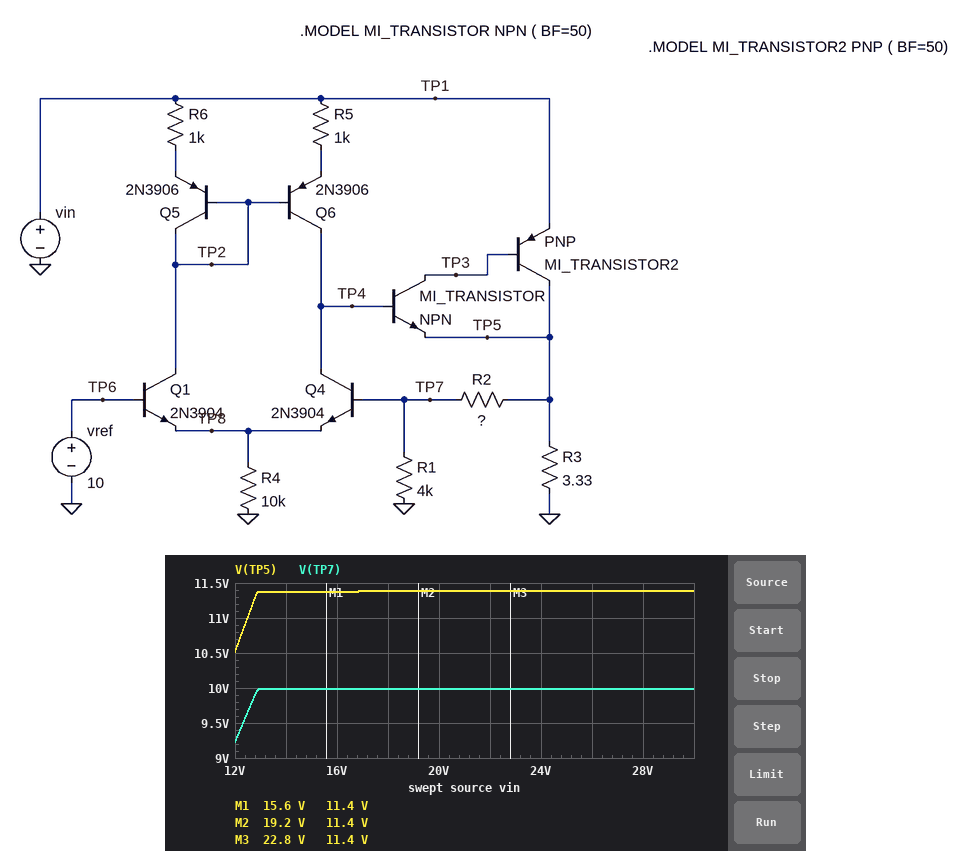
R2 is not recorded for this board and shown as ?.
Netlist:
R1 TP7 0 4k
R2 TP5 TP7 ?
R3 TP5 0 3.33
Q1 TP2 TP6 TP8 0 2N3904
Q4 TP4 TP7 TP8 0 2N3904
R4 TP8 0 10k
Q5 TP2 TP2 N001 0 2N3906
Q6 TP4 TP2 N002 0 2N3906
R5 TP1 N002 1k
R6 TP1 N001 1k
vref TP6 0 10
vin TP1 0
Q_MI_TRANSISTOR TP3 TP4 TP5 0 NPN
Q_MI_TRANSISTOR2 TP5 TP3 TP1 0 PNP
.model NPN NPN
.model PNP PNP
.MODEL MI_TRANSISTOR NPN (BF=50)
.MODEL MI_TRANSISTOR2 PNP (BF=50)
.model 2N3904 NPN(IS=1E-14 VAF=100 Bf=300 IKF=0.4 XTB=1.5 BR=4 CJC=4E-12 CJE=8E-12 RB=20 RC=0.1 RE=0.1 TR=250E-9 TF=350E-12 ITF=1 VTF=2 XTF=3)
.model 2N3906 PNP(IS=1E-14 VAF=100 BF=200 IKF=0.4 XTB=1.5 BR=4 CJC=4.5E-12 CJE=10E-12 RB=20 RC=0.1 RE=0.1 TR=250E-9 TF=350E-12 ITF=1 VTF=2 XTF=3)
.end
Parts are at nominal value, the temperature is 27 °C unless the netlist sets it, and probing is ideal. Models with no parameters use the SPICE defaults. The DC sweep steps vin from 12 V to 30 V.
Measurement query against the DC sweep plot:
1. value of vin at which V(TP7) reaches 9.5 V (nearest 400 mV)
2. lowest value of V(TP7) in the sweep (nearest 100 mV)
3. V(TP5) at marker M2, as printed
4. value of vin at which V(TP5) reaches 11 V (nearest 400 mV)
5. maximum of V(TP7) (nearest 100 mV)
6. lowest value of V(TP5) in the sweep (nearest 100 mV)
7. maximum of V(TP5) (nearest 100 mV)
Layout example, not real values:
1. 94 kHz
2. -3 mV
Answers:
1. 12.4 V
2. 9.2 V
3. 11.4 V
4. 12.4 V
5. 10.0 V
6. 10.5 V
7. 11.4 V
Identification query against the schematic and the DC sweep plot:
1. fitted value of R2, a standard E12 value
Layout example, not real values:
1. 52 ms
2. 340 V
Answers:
1. 560 Ω
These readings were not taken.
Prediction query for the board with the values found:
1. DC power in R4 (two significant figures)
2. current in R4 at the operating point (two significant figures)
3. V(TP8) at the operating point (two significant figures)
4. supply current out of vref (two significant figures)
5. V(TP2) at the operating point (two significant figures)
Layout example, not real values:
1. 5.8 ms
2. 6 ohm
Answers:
1. 8.6 mW
2. 930 µA
3. 9.3 V
4. 930 µA
5. 9.3 V
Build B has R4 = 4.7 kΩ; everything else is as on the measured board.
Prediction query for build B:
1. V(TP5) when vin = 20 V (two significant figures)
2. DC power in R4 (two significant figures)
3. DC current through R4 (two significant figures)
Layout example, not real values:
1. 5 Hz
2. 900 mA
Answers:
1. 11 V
2. 18 mW
3. 2.0 mA
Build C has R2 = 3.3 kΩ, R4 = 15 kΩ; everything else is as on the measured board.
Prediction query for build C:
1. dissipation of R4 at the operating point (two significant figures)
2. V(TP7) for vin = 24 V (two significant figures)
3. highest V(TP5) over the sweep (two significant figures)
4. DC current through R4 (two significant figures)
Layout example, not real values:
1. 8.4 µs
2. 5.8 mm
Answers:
1. 5.8 mW
2. 9.9 V
3. 18 V
4. 620 µA
